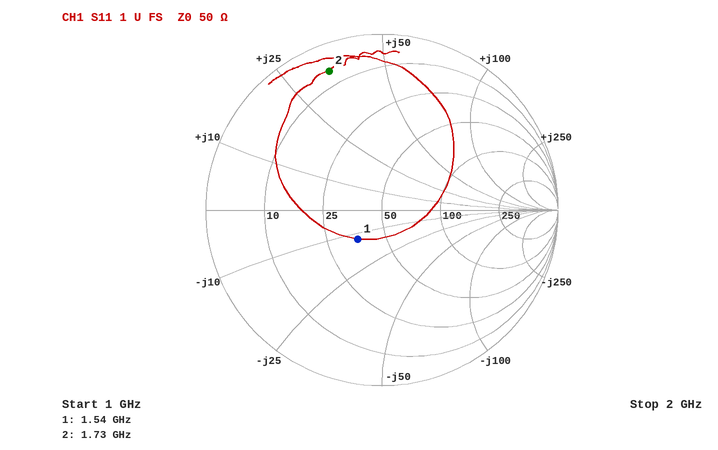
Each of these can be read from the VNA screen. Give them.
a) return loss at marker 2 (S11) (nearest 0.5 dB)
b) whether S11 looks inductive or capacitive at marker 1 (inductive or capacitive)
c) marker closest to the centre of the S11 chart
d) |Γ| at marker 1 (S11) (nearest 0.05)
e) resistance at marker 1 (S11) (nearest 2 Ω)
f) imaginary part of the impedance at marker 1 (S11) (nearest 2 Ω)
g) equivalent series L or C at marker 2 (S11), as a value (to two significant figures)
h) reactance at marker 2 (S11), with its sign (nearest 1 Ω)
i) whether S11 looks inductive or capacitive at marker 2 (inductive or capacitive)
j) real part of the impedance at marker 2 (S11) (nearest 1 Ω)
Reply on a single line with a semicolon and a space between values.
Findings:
1.5 dB; capacitive; marker 1; 0.20; 36 Ω; -12 Ω; 3.1 nH; +34 Ω; inductive; 6 Ω
